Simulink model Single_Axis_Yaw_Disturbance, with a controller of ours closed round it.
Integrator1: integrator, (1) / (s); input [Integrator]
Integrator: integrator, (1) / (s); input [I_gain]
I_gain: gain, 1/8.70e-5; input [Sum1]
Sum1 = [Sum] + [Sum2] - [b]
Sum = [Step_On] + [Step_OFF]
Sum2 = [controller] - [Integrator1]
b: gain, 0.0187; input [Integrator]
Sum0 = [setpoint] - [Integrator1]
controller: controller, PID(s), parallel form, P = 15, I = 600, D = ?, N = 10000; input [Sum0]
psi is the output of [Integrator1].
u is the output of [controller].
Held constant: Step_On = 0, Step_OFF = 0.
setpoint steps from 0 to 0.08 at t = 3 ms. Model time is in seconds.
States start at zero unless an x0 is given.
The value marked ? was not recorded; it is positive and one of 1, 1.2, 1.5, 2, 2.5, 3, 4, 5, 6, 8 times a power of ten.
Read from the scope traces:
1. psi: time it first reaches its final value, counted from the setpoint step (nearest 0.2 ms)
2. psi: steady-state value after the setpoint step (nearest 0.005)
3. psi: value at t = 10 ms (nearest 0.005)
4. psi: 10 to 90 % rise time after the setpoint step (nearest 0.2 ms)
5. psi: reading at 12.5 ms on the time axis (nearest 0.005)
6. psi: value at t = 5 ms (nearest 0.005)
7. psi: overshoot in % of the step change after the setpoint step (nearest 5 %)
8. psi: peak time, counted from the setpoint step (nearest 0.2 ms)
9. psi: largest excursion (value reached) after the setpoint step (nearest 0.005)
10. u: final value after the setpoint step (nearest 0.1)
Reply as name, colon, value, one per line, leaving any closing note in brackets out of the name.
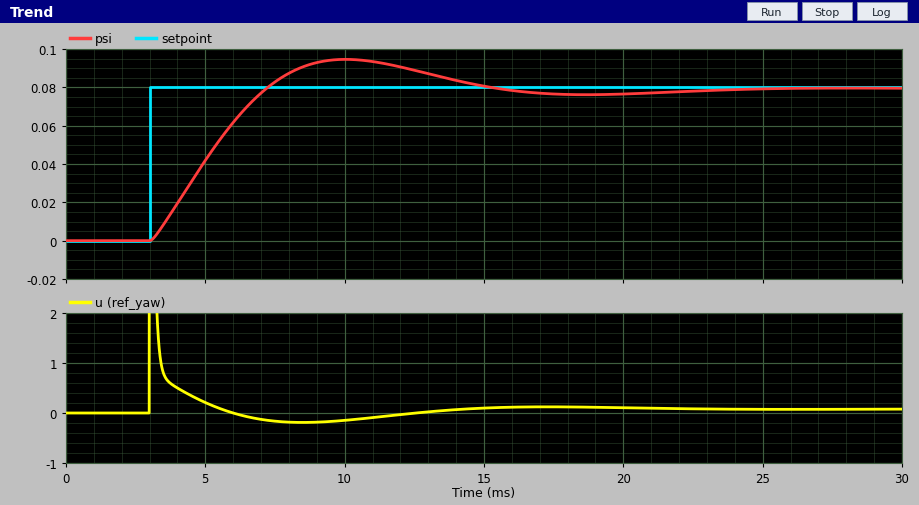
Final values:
psi: time it first reaches its final value, counted from the setpoint step: 4.2 ms
psi: steady-state value after the setpoint step: 0.080
psi: value at t = 10 ms: 0.095
psi: 10 to 90 % rise time after the setpoint step: 3.2 ms
psi: reading at 12.5 ms on the time axis: 0.090
psi: value at t = 5 ms: 0.040
psi: overshoot in % of the step change after the setpoint step: 20 %
psi: peak time, counted from the setpoint step: 7.0 ms
psi: largest excursion (value reached) after the setpoint step: 0.095
u: final value after the setpoint step: 0.1
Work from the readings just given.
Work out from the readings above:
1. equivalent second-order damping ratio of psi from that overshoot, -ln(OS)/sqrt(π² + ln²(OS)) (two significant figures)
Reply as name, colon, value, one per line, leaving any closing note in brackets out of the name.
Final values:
equivalent second-order damping ratio of psi from that overshoot, -ln(OS)/sqrt(π² + ln²(OS)): 0.46
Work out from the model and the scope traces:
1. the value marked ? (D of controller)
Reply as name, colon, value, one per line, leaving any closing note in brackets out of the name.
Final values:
the value marked ?: 0.02
